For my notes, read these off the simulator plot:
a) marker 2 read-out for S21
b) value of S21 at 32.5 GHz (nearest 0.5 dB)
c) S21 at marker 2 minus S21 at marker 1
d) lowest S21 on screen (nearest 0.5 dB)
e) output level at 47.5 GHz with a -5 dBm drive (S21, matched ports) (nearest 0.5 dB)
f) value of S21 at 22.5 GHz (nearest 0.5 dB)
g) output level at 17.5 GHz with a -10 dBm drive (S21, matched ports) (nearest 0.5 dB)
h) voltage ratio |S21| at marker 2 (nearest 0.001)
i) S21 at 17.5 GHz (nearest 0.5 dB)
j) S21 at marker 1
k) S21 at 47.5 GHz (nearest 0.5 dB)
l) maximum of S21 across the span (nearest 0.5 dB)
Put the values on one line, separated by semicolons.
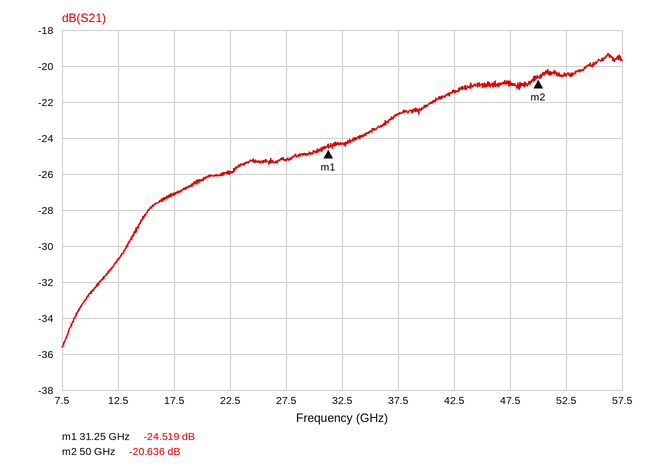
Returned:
-20.636 dB; -24.5 dB; 3.883 dB; -35.5 dB; -26.0 dBm; -26.0 dB; -37.0 dBm; 0.093; -27.0 dB; -24.519 dB; -21.0 dB; -19.5 dB
